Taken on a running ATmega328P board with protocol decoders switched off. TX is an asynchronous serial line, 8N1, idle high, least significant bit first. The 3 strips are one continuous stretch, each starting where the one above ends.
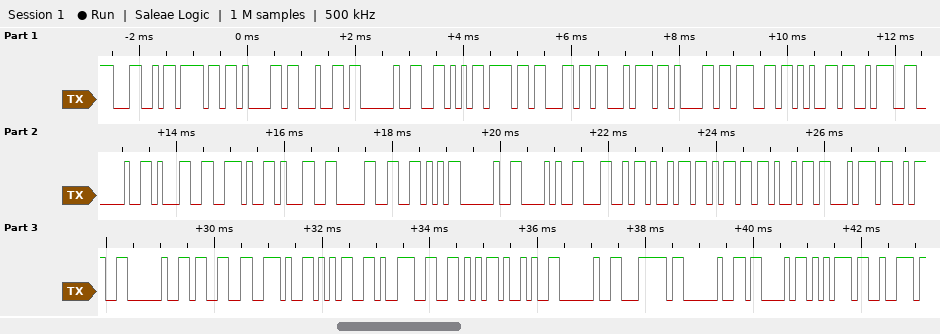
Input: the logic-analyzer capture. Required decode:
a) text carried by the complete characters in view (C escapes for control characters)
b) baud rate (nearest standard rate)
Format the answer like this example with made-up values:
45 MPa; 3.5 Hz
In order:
"Load Voltage: 1.10V (Limit: 3.59V) | Cur"; 9600 baud
